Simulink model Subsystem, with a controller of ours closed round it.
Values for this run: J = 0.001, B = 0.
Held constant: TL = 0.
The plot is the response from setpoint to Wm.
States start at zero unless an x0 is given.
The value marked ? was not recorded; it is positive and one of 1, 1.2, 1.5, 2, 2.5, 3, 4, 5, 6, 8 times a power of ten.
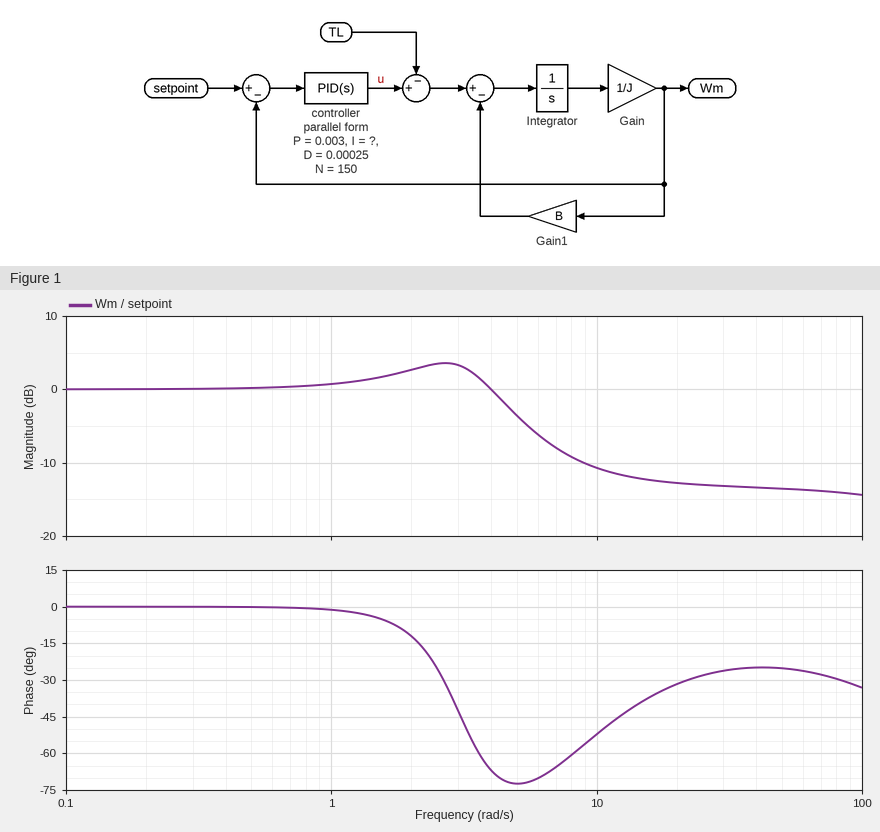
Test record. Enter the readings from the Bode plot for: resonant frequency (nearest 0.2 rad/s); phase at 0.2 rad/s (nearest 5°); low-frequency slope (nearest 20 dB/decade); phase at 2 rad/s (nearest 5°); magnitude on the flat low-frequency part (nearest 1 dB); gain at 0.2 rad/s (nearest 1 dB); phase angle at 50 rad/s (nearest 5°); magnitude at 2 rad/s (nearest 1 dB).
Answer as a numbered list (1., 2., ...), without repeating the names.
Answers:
1. 2.6 rad/s
2. 0°
3. 0 dB/decade
4. -10°
5. 0 dB
6. 0 dB
7. -25°
8. 3 dB
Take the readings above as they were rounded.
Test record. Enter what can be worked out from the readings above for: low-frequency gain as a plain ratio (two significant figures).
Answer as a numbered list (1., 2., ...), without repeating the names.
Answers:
1. 1.0
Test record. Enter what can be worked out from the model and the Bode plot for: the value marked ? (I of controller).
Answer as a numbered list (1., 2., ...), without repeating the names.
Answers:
1. 0.012
